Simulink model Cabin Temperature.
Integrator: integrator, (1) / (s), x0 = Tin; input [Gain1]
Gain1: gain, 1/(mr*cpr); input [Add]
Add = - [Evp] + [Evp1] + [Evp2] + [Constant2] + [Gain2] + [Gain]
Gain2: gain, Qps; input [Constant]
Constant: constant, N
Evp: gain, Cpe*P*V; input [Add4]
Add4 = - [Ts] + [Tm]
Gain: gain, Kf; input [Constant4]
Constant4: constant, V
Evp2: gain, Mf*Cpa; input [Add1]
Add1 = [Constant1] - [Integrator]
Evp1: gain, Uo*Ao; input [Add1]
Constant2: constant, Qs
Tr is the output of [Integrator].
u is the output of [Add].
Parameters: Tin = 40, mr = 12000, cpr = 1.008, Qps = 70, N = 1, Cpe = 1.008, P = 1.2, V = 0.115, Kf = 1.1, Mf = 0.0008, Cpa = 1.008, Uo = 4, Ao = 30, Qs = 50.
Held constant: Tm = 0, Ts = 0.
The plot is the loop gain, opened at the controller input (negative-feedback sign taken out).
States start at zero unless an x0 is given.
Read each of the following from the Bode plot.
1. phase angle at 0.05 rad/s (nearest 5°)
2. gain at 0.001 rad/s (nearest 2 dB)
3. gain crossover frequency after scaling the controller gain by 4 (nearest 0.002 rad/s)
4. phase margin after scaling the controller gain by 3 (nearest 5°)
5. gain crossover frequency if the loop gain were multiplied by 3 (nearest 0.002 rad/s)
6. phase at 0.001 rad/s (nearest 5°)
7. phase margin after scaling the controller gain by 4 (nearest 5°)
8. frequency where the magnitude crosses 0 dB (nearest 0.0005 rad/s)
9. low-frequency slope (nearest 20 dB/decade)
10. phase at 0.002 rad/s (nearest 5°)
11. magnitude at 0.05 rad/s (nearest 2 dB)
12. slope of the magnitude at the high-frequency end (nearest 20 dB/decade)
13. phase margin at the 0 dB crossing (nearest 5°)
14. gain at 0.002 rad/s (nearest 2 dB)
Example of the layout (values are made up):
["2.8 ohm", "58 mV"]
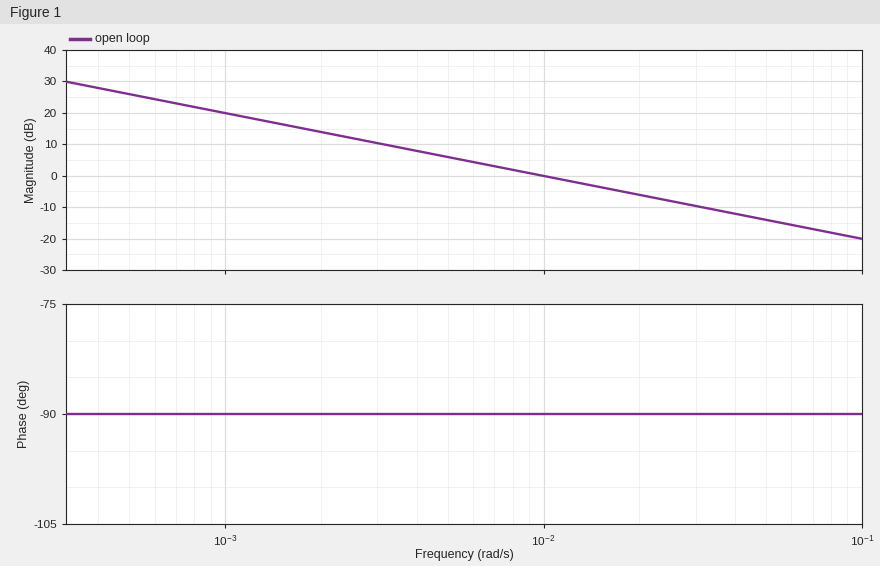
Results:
["-90°", "20 dB", "0.040 rad/s", "90°", "0.030 rad/s", "-90°", "90°", "0.0100 rad/s", "-20 dB/decade", "-90°", "-14 dB", "-20 dB/decade", "90°", "14 dB"]
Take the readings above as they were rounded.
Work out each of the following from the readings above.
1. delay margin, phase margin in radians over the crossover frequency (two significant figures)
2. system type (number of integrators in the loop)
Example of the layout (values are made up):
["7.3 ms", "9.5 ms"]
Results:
["160 s", "1"]
